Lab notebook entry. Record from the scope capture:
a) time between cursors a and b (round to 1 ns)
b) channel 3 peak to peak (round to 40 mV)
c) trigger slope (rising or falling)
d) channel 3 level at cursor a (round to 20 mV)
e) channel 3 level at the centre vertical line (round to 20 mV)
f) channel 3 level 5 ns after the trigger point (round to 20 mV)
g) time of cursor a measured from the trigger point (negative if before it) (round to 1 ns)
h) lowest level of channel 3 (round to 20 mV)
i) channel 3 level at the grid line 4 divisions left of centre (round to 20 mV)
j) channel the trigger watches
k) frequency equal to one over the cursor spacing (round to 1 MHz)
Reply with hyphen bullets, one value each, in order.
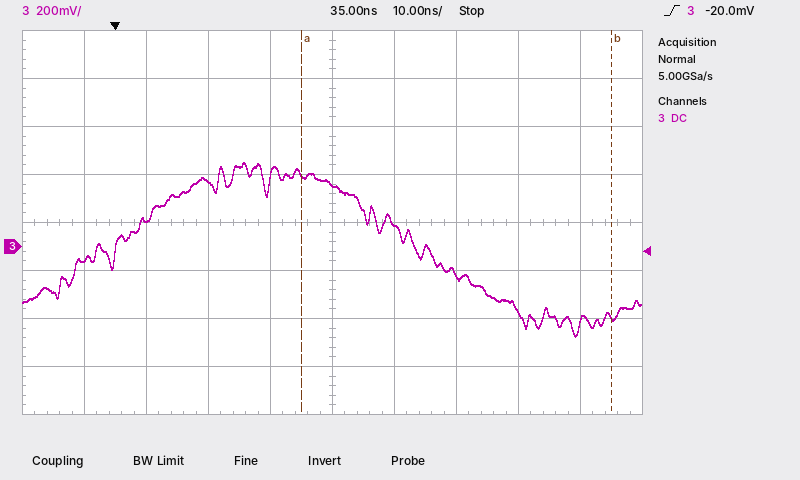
- 50 ns
- 720 mV
- rising
- 300 mV
- 260 mV
- 120 mV
- +30 ns
- -380 mV
- -60 mV
- channel 3
- 20 MHz
